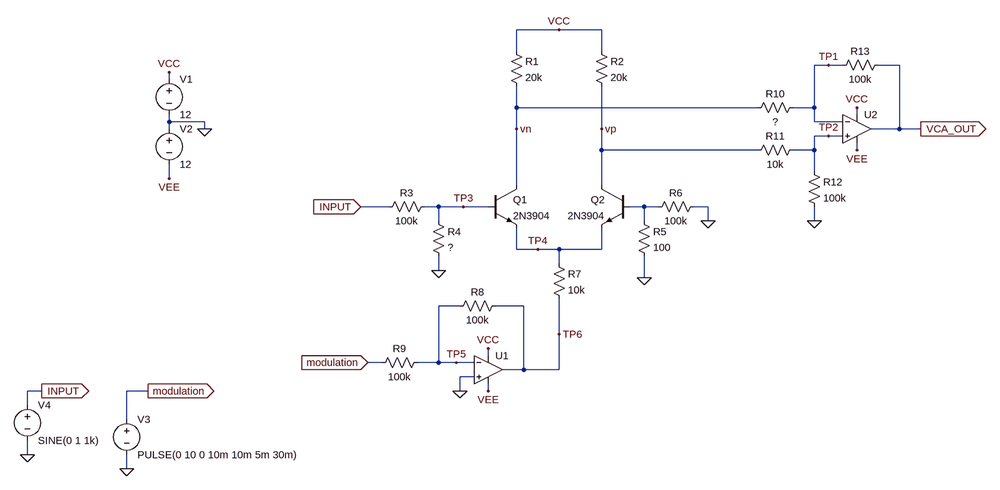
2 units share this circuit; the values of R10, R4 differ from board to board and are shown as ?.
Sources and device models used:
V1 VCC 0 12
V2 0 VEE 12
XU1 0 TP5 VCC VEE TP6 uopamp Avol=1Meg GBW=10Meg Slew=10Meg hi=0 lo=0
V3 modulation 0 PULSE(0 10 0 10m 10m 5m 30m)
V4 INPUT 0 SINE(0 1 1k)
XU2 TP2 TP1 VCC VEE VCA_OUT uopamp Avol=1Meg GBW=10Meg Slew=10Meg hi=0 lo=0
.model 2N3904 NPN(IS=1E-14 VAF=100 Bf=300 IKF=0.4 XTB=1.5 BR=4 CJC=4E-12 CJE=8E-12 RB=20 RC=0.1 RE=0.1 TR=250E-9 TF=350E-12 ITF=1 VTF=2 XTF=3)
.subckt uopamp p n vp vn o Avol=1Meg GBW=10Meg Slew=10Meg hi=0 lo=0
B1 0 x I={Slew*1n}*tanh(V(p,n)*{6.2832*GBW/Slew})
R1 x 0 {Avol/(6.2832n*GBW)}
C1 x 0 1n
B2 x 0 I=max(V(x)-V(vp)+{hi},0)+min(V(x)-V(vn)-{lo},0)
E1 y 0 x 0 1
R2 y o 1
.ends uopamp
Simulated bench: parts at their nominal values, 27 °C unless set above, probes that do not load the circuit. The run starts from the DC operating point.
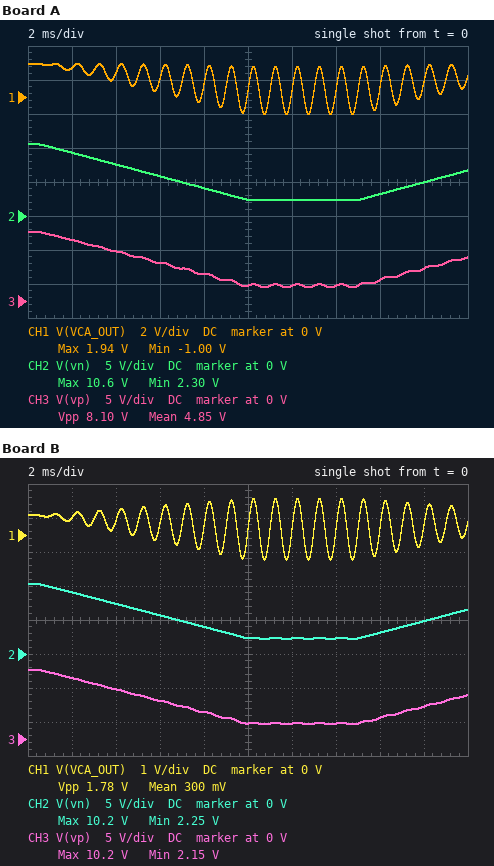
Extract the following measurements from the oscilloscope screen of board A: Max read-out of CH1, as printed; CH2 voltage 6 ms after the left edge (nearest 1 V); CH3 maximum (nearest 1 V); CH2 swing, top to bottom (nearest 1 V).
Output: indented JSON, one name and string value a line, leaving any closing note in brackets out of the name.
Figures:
{
  "Max read-out of CH1, as printed": "1.94 V",
  "CH2 voltage 6 ms after the left edge": "6 V",
  "CH3 maximum": "10 V",
  "CH2 swing, top to bottom": "8 V"
}
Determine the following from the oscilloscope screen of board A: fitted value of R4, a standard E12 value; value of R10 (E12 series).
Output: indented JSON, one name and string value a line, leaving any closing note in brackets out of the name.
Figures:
{
  "fitted value of R4, a standard E12 value": "150 Ω",
  "value of R10": "18 kΩ"
}
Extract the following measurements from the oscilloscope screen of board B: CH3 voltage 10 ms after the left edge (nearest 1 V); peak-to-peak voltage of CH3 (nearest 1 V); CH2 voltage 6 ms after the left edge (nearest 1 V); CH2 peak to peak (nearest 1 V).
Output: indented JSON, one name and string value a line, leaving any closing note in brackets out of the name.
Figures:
{
  "CH3 voltage 10 ms after the left edge": "2 V",
  "peak-to-peak voltage of CH3": "8 V",
  "CH2 voltage 6 ms after the left edge": "6 V",
  "CH2 peak to peak": "8 V"
}
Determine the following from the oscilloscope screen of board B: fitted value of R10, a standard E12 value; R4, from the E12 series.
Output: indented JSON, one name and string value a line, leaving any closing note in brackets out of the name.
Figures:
{
  "fitted value of R10, a standard E12 value": "12 kΩ",
  "R4, from the E12 series": "82 Ω"
}
